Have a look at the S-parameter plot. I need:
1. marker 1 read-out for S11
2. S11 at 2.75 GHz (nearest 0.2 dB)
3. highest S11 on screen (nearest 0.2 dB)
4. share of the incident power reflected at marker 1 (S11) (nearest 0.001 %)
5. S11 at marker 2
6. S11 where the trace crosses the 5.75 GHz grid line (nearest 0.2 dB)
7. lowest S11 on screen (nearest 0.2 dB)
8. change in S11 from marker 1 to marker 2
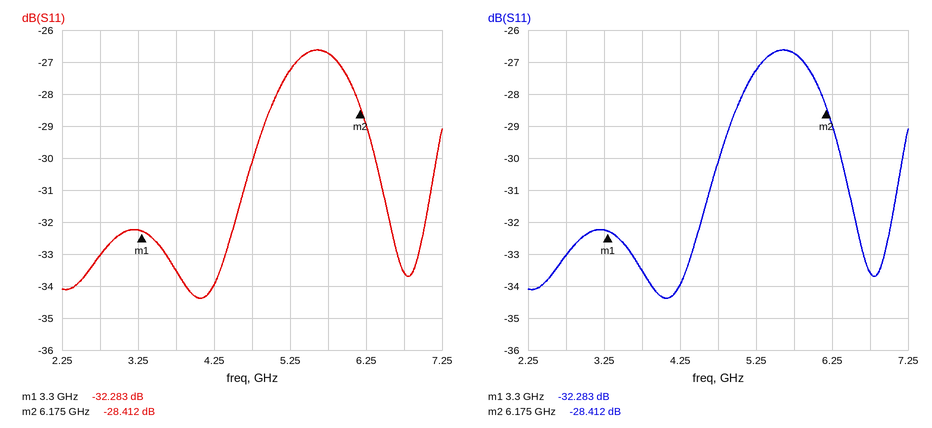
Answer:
-32.283 dB
-33.0 dB
-26.6 dB
0.059 %
-28.412 dB
-26.8 dB
-34.4 dB
3.871 dB
